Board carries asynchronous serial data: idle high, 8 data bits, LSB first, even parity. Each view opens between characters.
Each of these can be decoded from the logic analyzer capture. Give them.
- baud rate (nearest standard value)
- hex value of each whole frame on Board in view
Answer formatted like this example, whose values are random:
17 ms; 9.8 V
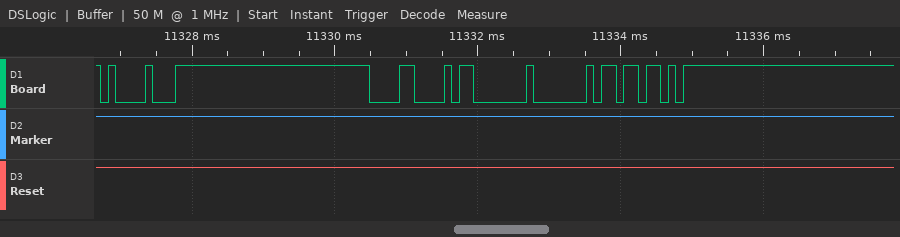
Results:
9600 baud; 21, 18, 03, 40, 5B
